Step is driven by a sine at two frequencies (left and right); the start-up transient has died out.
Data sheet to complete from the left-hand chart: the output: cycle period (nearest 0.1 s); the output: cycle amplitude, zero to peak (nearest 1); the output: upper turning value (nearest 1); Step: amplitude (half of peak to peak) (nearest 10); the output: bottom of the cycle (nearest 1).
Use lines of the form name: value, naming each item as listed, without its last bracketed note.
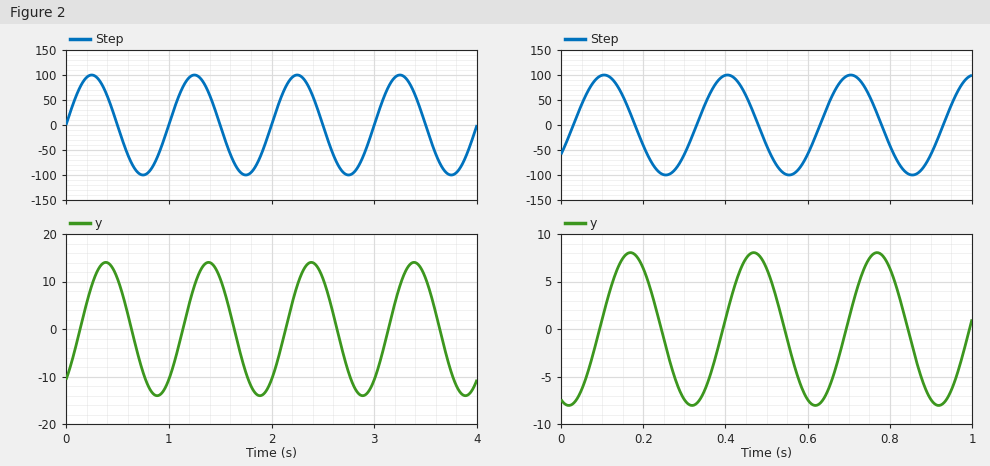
the output: cycle period: 1.0 s
the output: cycle amplitude, zero to peak: 14
the output: upper turning value: 14
Step: amplitude (half of peak to peak): 100
the output: bottom of the cycle: -14
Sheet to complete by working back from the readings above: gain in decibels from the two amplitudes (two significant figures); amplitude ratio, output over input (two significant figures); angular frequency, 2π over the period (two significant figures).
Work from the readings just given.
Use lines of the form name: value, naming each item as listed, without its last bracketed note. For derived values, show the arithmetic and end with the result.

gain in decibels from the two amplitudes: 20 log10(14 / 100) = -17 dB
amplitude ratio, output over input: 14 / 100 = 0.14
angular frequency, 2π over the period: 2π / 1 = 6.3 rad/s
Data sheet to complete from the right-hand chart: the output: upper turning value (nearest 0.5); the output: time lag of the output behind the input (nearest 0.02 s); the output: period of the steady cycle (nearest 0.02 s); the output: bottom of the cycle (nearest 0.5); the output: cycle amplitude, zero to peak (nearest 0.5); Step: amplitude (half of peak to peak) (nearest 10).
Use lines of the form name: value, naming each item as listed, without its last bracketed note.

the output: upper turning value: 8.0
the output: time lag of the output behind the input: 0.06 s
the output: period of the steady cycle: 0.30 s
the output: bottom of the cycle: -8.0
the output: cycle amplitude, zero to peak: 8.0
Step: amplitude (half of peak to peak): 100
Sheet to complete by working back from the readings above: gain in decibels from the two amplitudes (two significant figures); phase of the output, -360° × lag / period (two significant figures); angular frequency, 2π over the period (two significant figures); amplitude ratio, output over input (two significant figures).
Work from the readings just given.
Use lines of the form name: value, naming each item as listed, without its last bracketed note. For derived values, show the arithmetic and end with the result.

gain in decibels from the two amplitudes: 20 log10(8 / 100) = -22 dB
phase of the output, -360° × lag / period: -360 × 0.06 / 0.3 = -72°
angular frequency, 2π over the period: 2π / 0.3 = 21 rad/s
amplitude ratio, output over input: 8 / 100 = 0.080
